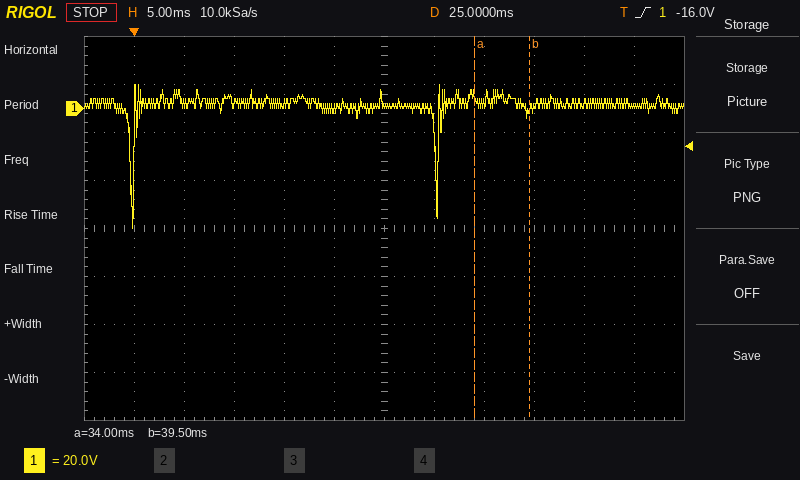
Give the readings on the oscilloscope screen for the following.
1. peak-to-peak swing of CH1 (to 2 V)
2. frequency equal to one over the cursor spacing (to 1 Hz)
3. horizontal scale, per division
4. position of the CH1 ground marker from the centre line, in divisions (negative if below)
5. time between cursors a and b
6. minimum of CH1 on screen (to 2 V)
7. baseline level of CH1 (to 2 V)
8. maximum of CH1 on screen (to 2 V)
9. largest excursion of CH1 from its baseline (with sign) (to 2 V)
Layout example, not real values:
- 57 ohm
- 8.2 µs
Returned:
- 60 V
- 182 Hz
- 5 ms
- +2.5 div
- 5.5 ms
- -50 V
- 2 V
- 10 V
- -52 V
